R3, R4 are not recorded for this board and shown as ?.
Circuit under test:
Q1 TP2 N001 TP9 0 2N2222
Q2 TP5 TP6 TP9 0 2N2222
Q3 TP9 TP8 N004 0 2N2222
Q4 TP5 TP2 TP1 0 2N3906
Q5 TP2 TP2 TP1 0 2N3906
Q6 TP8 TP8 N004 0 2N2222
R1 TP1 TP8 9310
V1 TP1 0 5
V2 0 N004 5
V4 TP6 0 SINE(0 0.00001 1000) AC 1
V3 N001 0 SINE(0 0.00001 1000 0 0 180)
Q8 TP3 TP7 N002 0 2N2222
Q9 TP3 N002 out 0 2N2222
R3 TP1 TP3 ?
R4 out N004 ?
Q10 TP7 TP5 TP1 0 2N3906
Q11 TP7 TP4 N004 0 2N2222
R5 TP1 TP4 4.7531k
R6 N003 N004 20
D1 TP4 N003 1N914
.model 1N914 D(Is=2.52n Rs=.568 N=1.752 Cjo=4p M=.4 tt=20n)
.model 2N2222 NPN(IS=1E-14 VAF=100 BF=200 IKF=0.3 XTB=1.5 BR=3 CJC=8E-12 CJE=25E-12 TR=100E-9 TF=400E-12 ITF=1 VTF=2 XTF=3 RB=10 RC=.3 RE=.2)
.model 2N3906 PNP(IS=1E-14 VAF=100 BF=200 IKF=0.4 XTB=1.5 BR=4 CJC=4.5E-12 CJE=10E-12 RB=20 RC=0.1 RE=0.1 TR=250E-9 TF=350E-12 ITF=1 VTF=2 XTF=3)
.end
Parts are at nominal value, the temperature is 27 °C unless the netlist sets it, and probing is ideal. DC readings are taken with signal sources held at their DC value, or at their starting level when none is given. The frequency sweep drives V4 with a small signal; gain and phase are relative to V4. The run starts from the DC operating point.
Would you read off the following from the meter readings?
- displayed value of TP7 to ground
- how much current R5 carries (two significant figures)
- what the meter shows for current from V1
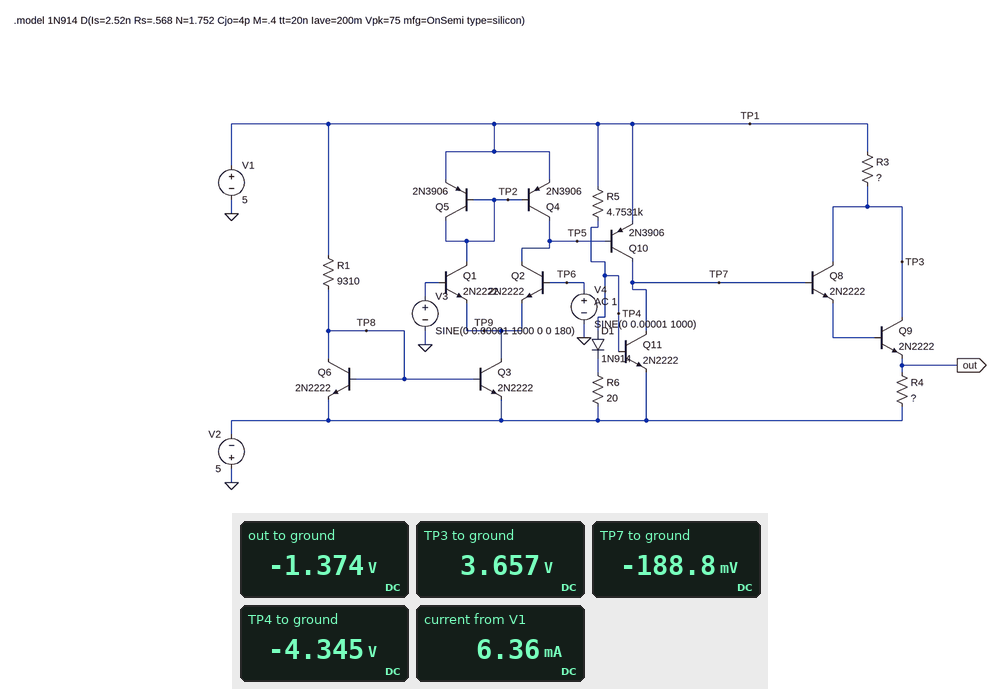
-188.8 mV
2.0 mA
6.36 mA
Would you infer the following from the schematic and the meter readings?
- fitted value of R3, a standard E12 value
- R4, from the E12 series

1 kΩ
2.7 kΩ
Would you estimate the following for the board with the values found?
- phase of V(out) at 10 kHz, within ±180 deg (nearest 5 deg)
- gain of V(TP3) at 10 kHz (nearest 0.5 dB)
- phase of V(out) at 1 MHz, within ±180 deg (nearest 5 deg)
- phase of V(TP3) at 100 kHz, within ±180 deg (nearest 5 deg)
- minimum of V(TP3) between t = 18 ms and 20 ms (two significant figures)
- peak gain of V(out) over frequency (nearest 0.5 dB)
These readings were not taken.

-60 deg
91.5 dB
-100 deg
90 deg
2.5 V
106.0 dB
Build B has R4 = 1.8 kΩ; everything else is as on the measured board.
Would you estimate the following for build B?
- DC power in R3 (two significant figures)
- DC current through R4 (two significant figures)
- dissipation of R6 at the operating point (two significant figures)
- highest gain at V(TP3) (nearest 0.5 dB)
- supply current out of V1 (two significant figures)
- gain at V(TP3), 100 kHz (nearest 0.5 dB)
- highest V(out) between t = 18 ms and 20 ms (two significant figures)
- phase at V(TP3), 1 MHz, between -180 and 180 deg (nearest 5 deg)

4.0 mW
2.0 mA
77 µW
100.5 dB
7.0 mA
76.5 dB
1.0 V
75 deg
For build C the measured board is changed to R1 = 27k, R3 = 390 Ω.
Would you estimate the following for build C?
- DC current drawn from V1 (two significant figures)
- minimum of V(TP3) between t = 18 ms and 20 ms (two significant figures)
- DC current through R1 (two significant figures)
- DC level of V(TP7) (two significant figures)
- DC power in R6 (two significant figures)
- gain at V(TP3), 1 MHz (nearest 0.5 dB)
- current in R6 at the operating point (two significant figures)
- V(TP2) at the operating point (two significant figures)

3.0 mA
5.0 V
350 µA
-5.0 V
69 µW
-14.0 dB
1.9 mA
4.4 V
